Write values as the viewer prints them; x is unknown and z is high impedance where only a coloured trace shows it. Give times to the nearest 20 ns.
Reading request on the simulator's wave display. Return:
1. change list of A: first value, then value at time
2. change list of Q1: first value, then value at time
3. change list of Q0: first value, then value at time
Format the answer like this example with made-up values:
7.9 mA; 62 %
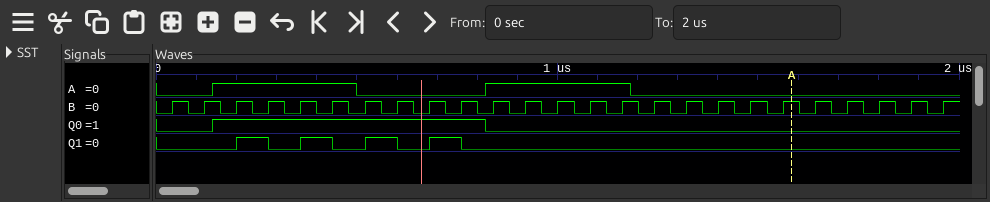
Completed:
0, 1 at 140 ns, 0 at 500 ns, 1 at 820 ns, 0 at 1180 ns; 0, 1 at 200 ns, 0 at 280 ns, 1 at 360 ns, 0 at 440 ns, 1 at 520 ns, 0 at 600 ns, 1 at 680 ns, 0 at 760 ns; 0, 1 at 140 ns, 0 at 820 ns
